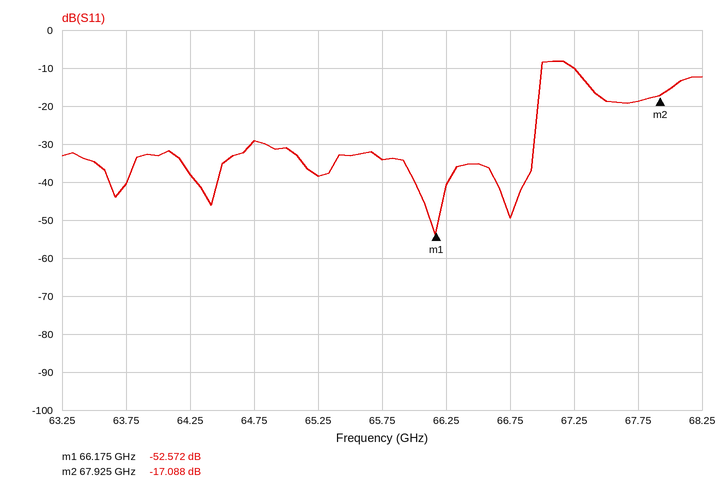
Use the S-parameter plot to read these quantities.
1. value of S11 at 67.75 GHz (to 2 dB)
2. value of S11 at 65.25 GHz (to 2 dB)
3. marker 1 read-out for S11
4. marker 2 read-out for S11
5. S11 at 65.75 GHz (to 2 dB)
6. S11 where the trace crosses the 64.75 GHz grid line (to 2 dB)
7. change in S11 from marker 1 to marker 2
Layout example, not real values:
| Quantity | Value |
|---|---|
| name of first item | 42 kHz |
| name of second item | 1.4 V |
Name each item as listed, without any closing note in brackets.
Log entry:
| Quantity | Value |
|---|---|
| value of S11 at 67.75 GHz | -18 dB |
| value of S11 at 65.25 GHz | -38 dB |
| marker 1 read-out for S11 | -52.572 dB |
| marker 2 read-out for S11 | -17.088 dB |
| S11 at 65.75 GHz | -34 dB |
| S11 where the trace crosses the 64.75 GHz grid line | -30 dB |
| change in S11 from marker 1 to marker 2 | 35.484 dB |
